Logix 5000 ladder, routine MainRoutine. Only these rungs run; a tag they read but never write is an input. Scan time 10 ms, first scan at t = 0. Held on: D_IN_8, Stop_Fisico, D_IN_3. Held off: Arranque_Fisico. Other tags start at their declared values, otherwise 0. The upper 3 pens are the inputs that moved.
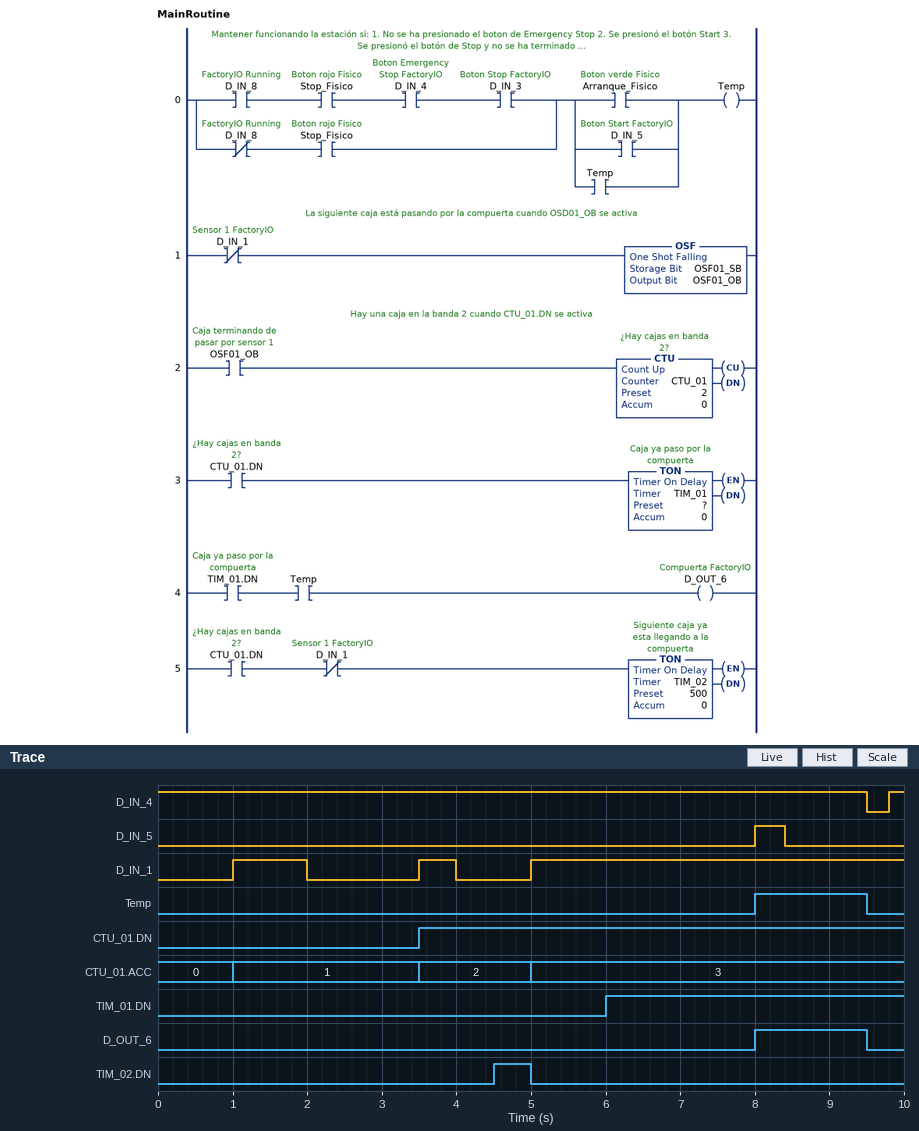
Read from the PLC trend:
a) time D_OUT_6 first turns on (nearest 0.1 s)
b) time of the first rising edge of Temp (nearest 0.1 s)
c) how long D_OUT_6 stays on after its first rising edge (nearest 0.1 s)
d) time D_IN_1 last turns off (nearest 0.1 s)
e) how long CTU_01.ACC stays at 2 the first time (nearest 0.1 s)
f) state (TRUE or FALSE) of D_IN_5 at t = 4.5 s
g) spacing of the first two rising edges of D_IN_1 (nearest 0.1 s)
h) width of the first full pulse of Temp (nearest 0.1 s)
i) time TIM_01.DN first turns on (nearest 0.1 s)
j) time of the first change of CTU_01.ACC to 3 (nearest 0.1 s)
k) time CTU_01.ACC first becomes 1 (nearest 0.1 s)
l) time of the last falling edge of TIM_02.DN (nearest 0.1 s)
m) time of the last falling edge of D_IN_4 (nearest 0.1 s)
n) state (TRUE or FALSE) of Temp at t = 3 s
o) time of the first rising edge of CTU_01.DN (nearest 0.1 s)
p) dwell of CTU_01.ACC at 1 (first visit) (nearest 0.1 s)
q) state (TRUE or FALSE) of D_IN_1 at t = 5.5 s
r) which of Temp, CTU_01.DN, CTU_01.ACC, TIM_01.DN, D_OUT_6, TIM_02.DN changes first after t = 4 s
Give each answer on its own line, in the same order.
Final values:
8.0 s
8.0 s
1.5 s
4.0 s
1.5 s
FALSE
2.5 s
1.5 s
6.0 s
5.0 s
1.0 s
5.0 s
9.5 s
FALSE
3.5 s
2.5 s
TRUE
TIM_02.DN
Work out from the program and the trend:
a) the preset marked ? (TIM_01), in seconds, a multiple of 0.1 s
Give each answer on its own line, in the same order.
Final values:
2.5 s
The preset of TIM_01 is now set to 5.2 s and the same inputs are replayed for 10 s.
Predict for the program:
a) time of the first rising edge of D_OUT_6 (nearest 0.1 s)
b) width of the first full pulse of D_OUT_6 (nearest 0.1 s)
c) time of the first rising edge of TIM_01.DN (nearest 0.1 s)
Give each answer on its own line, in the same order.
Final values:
8.7 s
0.8 s
8.7 s
